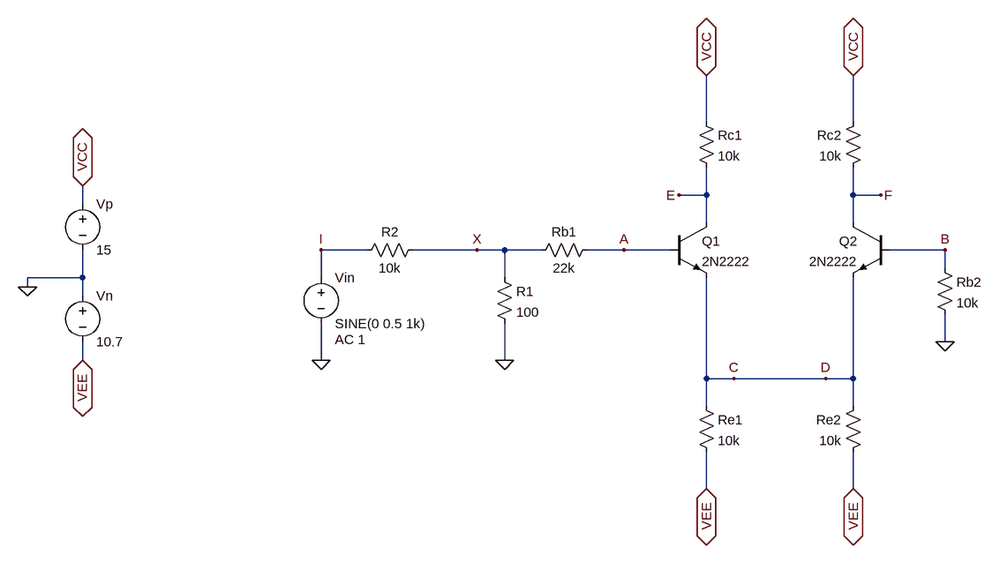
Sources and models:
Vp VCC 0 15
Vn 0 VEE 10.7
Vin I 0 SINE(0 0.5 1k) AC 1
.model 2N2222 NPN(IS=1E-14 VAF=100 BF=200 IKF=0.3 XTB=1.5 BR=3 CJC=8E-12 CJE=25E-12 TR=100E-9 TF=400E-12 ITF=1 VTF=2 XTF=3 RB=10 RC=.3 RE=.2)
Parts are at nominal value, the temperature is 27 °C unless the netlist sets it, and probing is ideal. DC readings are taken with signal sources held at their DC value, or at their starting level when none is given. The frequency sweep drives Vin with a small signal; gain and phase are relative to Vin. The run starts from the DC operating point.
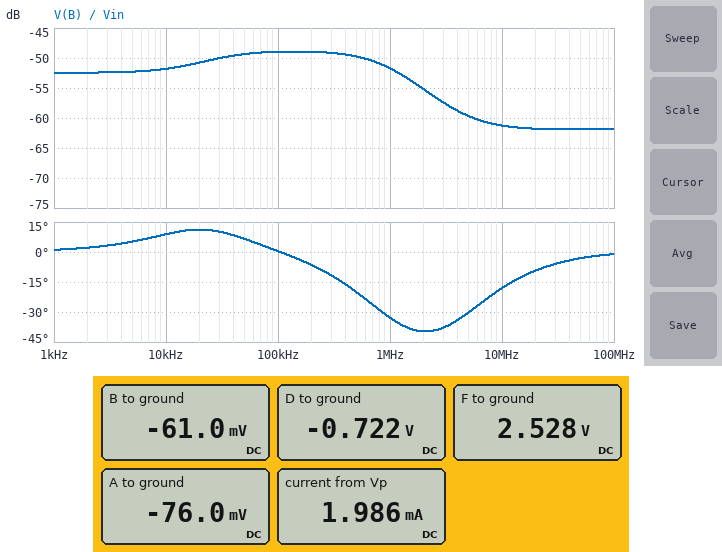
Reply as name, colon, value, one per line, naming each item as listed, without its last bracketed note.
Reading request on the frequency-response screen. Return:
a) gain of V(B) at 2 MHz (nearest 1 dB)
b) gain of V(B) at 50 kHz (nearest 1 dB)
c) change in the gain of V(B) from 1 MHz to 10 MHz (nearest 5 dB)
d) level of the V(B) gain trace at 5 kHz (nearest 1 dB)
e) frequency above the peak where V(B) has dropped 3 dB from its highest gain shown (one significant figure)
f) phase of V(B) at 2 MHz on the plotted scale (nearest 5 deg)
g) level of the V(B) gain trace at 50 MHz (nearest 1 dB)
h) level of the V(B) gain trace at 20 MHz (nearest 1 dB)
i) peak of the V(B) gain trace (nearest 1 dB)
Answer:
gain of V(B) at 2 MHz: -55 dB
gain of V(B) at 50 kHz: -49 dB
change in the gain of V(B) from 1 MHz to 10 MHz: -10 dB
level of the V(B) gain trace at 5 kHz: -52 dB
frequency above the peak where V(B) has dropped 3 dB from its highest gain shown: 1 MHz
phase of V(B) at 2 MHz on the plotted scale: -40 deg
level of the V(B) gain trace at 50 MHz: -62 dB
level of the V(B) gain trace at 20 MHz: -62 dB
peak of the V(B) gain trace: -49 dB
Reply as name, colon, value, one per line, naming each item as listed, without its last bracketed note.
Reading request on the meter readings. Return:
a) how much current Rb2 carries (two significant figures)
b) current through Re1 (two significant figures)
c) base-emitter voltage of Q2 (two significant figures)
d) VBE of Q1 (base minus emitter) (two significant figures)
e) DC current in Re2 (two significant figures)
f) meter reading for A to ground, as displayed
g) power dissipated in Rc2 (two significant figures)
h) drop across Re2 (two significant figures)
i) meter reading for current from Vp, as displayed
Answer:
how much current Rb2 carries: 6.1 µA
current through Re1: 1.0 mA
base-emitter voltage of Q2: 660 mV
VBE of Q1 (base minus emitter): 650 mV
DC current in Re2: 1.0 mA
meter reading for A to ground, as displayed: -76.0 mV
power dissipated in Rc2: 16 mW
drop across Re2: 10 V
meter reading for current from Vp, as displayed: 1.986 mA
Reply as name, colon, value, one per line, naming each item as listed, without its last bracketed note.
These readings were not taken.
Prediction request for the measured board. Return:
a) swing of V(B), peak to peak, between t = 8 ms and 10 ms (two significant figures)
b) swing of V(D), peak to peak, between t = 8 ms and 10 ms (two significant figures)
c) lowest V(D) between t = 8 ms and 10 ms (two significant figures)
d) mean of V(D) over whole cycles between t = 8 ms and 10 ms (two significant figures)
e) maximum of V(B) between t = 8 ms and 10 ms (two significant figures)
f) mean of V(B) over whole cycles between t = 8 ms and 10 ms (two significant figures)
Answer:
swing of V(B), peak to peak, between t = 8 ms and 10 ms: 2.4 mV
swing of V(D), peak to peak, between t = 8 ms and 10 ms: 3.4 mV
lowest V(D) between t = 8 ms and 10 ms: -720 mV
mean of V(D) over whole cycles between t = 8 ms and 10 ms: -720 mV
maximum of V(B) between t = 8 ms and 10 ms: -60 mV
mean of V(B) over whole cycles between t = 8 ms and 10 ms: -61 mV
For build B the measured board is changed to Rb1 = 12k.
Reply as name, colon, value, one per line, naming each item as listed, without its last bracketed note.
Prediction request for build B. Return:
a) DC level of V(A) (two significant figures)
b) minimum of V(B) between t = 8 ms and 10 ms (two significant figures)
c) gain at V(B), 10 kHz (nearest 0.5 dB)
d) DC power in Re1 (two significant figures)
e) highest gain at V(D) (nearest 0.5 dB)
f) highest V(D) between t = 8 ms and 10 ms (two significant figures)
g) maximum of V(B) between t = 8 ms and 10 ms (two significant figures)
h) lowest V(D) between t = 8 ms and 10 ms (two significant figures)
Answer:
DC level of V(A): -54 mV
minimum of V(B) between t = 8 ms and 10 ms: -52 mV
gain at V(B), 10 kHz: -50.0 dB
DC power in Re1: 10 mW
highest gain at V(D): -47.0 dB
highest V(D) between t = 8 ms and 10 ms: -700 mV
maximum of V(B) between t = 8 ms and 10 ms: -49 mV
lowest V(D) between t = 8 ms and 10 ms: -710 mV
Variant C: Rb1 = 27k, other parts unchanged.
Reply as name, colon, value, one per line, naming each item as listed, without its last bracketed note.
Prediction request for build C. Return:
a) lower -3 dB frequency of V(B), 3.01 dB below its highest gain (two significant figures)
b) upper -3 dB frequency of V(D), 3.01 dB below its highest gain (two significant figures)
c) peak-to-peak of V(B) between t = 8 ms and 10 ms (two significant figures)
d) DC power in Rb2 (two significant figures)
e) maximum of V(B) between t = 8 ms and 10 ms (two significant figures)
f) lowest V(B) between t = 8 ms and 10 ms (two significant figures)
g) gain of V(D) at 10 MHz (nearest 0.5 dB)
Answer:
lower -3 dB frequency of V(B), 3.01 dB below its highest gain: 9.8 kHz
upper -3 dB frequency of V(D), 3.01 dB below its highest gain: 930 kHz
peak-to-peak of V(B) between t = 8 ms and 10 ms: 2.2 mV
DC power in Rb2: 420 nW
maximum of V(B) between t = 8 ms and 10 ms: -64 mV
lowest V(B) between t = 8 ms and 10 ms: -66 mV
gain of V(D) at 10 MHz: -63.0 dB
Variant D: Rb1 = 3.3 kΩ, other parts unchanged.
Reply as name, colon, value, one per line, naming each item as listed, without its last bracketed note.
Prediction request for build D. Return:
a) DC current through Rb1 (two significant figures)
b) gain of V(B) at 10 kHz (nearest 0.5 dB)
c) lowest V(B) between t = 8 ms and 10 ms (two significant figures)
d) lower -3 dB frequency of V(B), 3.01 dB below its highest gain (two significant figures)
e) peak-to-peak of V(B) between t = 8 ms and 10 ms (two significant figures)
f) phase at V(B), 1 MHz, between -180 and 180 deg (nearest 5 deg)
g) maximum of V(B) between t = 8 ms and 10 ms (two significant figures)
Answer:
DC current through Rb1: 6.1 µA
gain of V(B) at 10 kHz: -48.0 dB
lowest V(B) between t = 8 ms and 10 ms: -37 mV
lower -3 dB frequency of V(B), 3.01 dB below its highest gain: 21 kHz
peak-to-peak of V(B) between t = 8 ms and 10 ms: 3.8 mV
phase at V(B), 1 MHz, between -180 and 180 deg: -10 deg
maximum of V(B) between t = 8 ms and 10 ms: -33 mV
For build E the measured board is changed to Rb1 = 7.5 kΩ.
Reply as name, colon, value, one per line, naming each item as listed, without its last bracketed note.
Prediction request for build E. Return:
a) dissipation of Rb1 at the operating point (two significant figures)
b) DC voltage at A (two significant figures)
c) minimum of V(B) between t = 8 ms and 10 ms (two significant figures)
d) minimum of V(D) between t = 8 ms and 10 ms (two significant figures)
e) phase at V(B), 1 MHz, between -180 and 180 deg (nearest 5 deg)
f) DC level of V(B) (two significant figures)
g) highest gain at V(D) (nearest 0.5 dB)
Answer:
dissipation of Rb1 at the operating point: 200 nW
DC voltage at A: -39 mV
minimum of V(B) between t = 8 ms and 10 ms: -45 mV
minimum of V(D) between t = 8 ms and 10 ms: -700 mV
phase at V(B), 1 MHz, between -180 and 180 deg: -20 deg
DC level of V(B): -44 mV
highest gain at V(D): -45.5 dB
